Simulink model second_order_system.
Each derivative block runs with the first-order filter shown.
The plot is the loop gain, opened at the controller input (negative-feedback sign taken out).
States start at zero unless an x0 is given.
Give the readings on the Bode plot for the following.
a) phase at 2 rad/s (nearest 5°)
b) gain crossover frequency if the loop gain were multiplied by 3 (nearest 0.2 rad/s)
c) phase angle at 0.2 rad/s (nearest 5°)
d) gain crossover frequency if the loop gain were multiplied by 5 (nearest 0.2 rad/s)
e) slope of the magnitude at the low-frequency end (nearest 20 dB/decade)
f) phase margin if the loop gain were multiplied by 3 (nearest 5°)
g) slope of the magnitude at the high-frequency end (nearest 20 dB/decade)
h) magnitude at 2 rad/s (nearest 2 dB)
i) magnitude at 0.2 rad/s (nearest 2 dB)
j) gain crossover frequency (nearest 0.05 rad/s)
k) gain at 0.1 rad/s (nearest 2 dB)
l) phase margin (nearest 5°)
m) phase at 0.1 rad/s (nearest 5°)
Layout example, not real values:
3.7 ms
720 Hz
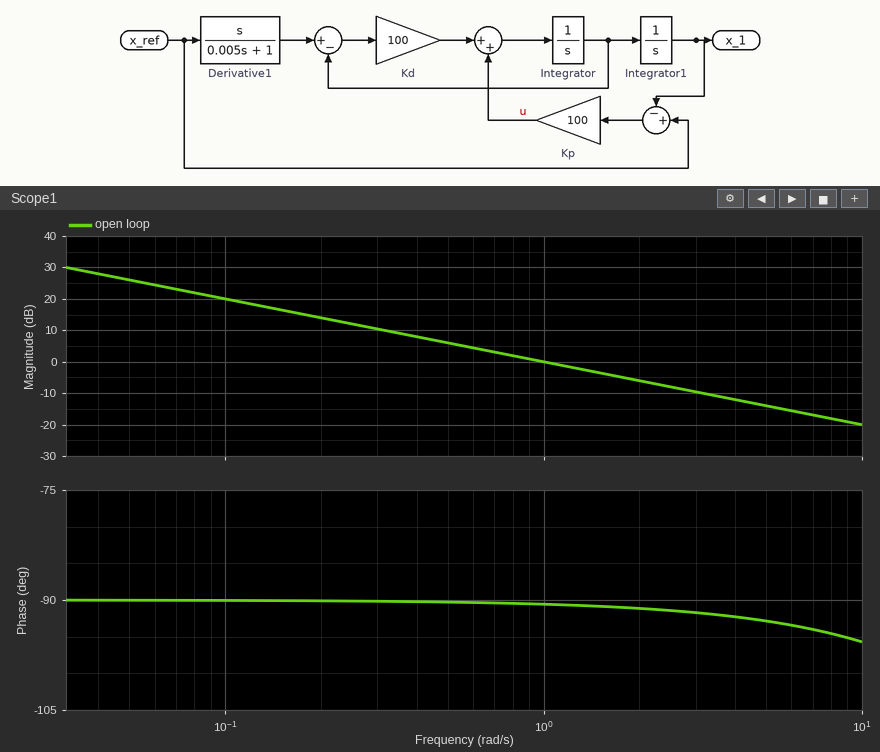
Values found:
-90°
3.0 rad/s
-90°
5.0 rad/s
-20 dB/decade
90°
-20 dB/decade
-6 dB
14 dB
1.00 rad/s
20 dB
90°
-90°
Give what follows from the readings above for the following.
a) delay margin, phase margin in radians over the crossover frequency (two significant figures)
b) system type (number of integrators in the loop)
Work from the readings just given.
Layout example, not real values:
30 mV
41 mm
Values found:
1.6 s
1
